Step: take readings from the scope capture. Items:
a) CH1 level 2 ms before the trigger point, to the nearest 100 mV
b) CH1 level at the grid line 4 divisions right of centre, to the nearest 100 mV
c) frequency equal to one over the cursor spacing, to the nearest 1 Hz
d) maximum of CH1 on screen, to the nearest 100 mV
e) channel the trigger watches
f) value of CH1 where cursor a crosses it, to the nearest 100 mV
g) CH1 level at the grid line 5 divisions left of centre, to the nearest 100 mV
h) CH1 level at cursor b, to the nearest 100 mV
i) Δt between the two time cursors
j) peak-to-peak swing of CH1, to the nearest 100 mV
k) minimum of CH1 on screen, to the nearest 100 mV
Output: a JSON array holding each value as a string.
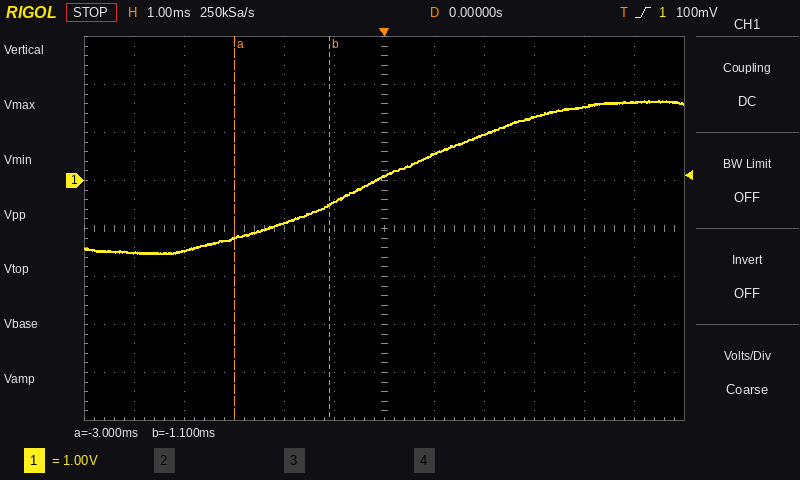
["-900 mV", "1.5 V", "526 Hz", "1.7 V", "CH1", "-1.2 V", "-1.5 V", "-500 mV", "1.9 ms", "3.2 V", "-1.5 V"]
